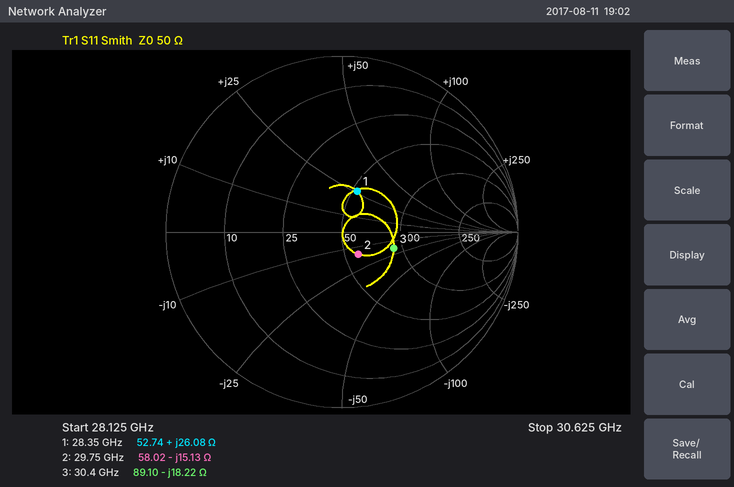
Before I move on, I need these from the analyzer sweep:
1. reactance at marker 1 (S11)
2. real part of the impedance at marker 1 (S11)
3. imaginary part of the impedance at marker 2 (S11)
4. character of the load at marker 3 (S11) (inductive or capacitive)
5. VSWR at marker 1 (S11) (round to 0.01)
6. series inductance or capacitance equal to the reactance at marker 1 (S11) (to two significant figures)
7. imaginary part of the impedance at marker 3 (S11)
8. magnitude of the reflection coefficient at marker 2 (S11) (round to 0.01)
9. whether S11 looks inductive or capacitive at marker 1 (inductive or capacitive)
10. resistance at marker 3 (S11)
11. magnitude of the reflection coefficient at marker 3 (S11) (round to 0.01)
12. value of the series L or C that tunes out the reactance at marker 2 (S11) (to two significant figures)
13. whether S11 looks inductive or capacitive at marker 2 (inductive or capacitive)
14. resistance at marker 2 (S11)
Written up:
+26.08 Ω
52.74 Ω
-15.13 Ω
capacitive
1.66
150 pH
-18.22 Ω
0.16
inductive
89.10 Ω
0.31
81 pH
capacitive
58.02 Ω
